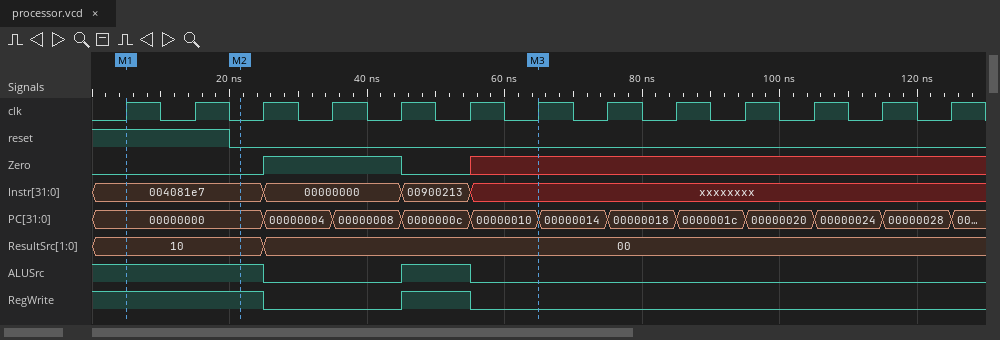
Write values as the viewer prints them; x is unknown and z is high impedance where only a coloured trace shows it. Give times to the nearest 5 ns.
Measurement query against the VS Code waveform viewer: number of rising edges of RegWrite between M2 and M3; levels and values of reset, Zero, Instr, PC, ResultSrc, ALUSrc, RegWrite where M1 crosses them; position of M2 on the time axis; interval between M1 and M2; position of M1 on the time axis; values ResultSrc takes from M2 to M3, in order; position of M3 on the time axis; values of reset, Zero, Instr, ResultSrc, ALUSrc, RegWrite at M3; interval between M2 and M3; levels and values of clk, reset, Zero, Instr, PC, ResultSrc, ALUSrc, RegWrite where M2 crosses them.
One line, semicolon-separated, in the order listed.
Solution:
1; reset=1, Zero=0, Instr=004081e7, PC=00000000, ResultSrc=10, ALUSrc=1, RegWrite=1; 20 ns; 15 ns; 5 ns; 10, 00; 65 ns; reset=0, Zero=x, Instr=xxxxxxxx, ResultSrc=00, ALUSrc=0, RegWrite=0; 45 ns; clk=0, reset=0, Zero=0, Instr=004081e7, PC=00000000, ResultSrc=10, ALUSrc=1, RegWrite=1
